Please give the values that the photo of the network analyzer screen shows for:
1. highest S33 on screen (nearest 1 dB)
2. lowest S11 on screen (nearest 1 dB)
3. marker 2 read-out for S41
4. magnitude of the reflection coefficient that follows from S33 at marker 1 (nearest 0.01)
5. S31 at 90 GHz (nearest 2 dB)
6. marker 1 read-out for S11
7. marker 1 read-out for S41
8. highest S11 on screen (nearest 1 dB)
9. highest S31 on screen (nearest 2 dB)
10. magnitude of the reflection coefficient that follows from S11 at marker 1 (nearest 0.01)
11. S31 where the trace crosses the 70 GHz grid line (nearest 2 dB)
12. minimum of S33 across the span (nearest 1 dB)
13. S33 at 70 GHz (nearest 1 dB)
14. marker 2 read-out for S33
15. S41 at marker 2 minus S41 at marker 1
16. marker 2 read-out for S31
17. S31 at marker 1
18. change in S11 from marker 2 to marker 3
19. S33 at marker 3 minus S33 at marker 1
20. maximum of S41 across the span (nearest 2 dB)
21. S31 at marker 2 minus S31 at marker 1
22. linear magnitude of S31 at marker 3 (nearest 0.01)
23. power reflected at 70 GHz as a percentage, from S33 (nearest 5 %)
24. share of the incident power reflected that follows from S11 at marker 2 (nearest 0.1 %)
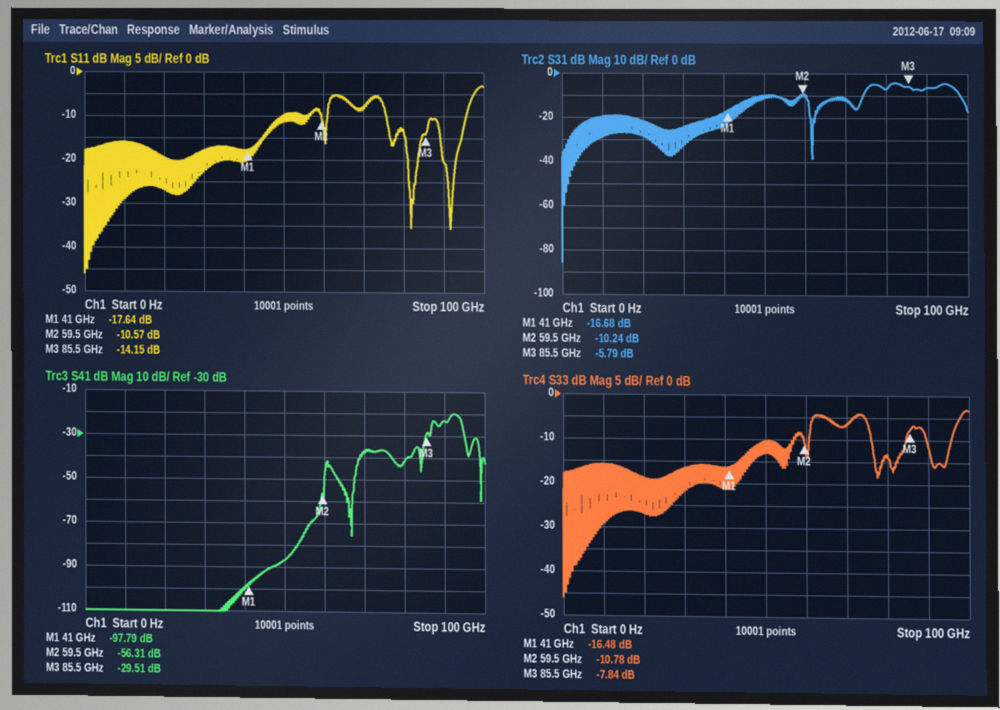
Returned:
-3 dB
-46 dB
-56.31 dB
0.15
-6 dB
-17.64 dB
-97.79 dB
-3 dB
-4 dB
0.13
-12 dB
-46 dB
-7 dB
-10.78 dB
41.48 dB
-10.24 dB
-16.68 dB
-3.58 dB
8.64 dB
-20 dB
6.44 dB
0.51
20 %
8.8 %
